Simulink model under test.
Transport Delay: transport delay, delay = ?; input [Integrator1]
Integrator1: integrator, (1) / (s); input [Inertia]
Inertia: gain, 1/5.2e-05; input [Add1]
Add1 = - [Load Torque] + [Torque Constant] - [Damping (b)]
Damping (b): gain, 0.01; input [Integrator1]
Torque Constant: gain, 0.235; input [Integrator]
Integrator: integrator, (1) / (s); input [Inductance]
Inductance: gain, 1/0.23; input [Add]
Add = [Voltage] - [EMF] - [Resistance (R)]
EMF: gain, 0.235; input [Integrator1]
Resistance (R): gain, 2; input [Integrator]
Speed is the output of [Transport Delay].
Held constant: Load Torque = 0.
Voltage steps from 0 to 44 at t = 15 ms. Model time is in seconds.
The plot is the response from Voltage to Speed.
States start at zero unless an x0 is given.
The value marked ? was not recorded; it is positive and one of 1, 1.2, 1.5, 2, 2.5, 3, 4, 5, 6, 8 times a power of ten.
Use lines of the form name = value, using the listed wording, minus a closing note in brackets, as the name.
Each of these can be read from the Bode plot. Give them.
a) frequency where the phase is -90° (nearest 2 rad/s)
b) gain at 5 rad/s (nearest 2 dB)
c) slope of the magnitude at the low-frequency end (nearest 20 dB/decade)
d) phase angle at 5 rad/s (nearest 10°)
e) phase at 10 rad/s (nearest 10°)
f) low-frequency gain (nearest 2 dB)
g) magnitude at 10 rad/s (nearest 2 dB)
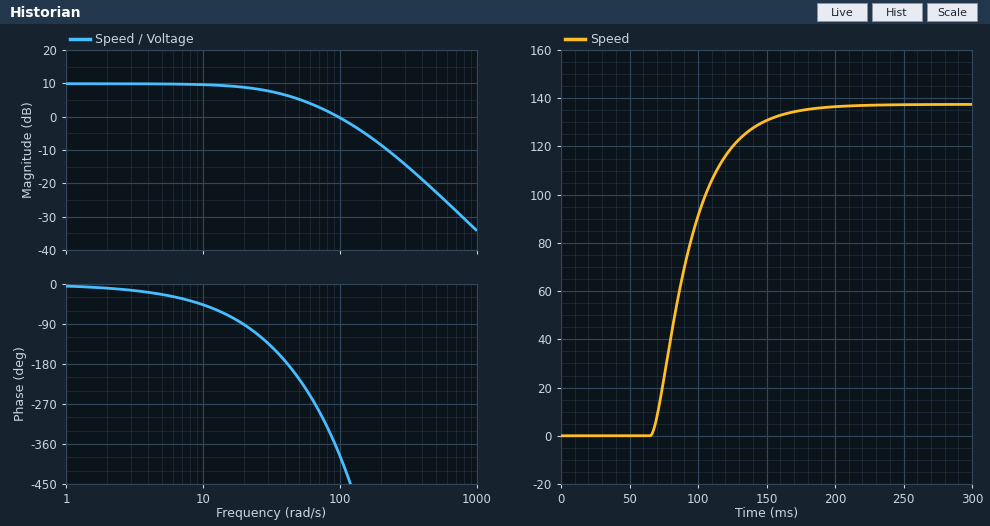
frequency where the phase is -90° = 20 rad/s
gain at 5 rad/s = 10 dB
slope of the magnitude at the low-frequency end = 0 dB/decade
phase angle at 5 rad/s = -20°
phase at 10 rad/s = -50°
low-frequency gain = 10 dB
magnitude at 10 rad/s = 10 dB
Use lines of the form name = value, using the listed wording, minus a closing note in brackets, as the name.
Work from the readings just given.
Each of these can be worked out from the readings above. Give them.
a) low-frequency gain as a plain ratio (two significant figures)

low-frequency gain as a plain ratio = 3.2
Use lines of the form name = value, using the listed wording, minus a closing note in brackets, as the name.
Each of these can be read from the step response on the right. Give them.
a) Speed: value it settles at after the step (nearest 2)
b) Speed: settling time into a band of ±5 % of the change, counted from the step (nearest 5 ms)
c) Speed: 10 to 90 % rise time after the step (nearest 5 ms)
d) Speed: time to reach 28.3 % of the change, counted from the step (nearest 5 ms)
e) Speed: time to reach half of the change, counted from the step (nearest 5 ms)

Speed: value it settles at after the step = 138
Speed: settling time into a band of ±5 % of the change, counted from the step = 135 ms
Speed: 10 to 90 % rise time after the step = 60 ms
Speed: time to reach 28.3 % of the change, counted from the step = 65 ms
Speed: time to reach half of the change, counted from the step = 75 ms
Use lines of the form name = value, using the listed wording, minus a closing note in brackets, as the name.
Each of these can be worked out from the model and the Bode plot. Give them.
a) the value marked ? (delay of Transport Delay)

the value marked ? = 0.05
